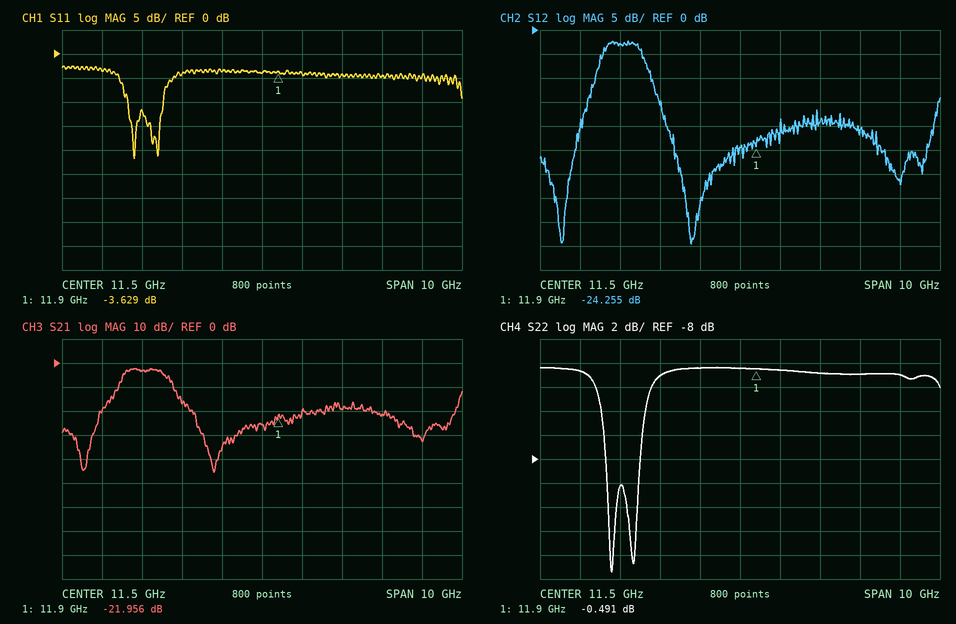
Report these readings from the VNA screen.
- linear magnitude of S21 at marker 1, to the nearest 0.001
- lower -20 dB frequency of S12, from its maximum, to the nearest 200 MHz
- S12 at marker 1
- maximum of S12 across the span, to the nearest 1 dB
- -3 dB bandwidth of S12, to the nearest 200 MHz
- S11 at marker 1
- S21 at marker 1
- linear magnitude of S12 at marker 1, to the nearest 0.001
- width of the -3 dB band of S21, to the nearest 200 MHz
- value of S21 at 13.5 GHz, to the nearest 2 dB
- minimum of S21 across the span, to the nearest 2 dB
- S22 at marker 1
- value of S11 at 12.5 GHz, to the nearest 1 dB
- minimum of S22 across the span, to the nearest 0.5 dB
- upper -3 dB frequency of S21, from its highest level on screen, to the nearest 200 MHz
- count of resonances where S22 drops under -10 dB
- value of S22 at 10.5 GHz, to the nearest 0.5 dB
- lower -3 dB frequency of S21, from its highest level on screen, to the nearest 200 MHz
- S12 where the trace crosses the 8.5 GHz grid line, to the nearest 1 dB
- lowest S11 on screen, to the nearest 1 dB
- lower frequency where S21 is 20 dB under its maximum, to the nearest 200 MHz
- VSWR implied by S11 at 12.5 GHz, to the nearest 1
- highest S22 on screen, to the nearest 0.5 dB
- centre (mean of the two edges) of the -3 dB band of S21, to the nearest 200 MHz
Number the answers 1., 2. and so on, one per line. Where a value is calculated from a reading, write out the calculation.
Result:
1. 10^(-21.956/20) ≈ 0.080
2. 7.4 GHz
3. -24.255 dB
4. -2 dB
5. 9.0 GHz − 8.0 GHz = 1.0 GHz
6. -3.629 dB
7. -21.956 dB
8. 10^(-24.255/20) ≈ 0.061
9. 9.0 GHz − 8.0 GHz = 1.0 GHz
10. -20 dB
11. -46 dB
12. -0.491 dB
13. -4 dB
14. -17.5 dB
15. 9.0 GHz
16. 2
17. -0.5 dB
18. 8.0 GHz
19. -3 dB
20. -22 dB
21. 7.4 GHz
22. |Γ| = 10^(-4/20) = 0.6310; VSWR = (1 + 0.6310)/(1 − 0.6310) ≈ 4
23. -0.5 dB
24. 8.6 GHz
